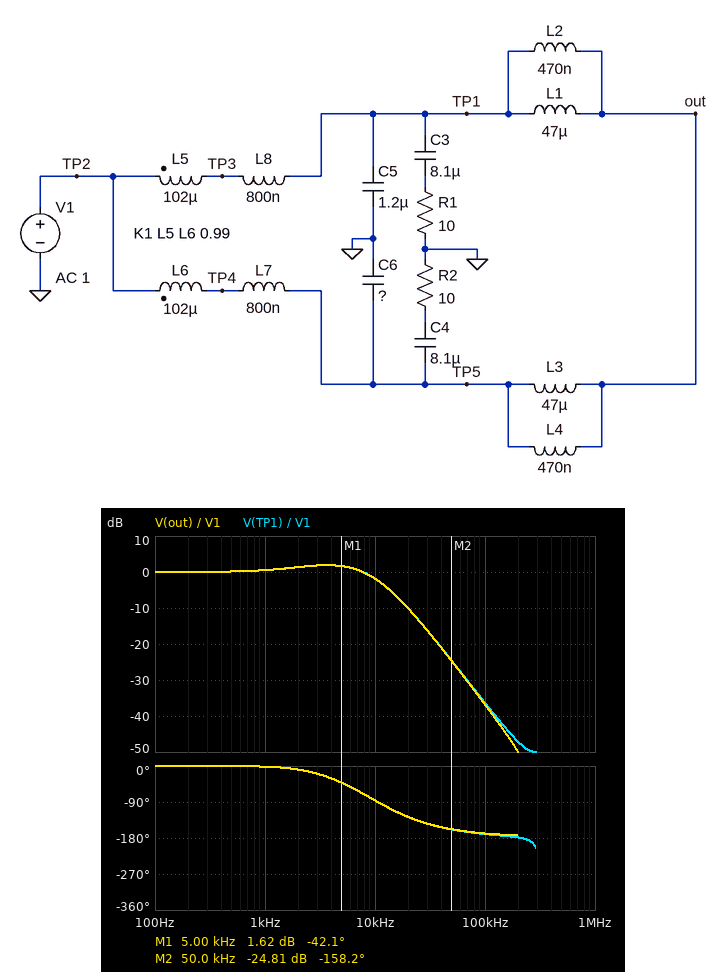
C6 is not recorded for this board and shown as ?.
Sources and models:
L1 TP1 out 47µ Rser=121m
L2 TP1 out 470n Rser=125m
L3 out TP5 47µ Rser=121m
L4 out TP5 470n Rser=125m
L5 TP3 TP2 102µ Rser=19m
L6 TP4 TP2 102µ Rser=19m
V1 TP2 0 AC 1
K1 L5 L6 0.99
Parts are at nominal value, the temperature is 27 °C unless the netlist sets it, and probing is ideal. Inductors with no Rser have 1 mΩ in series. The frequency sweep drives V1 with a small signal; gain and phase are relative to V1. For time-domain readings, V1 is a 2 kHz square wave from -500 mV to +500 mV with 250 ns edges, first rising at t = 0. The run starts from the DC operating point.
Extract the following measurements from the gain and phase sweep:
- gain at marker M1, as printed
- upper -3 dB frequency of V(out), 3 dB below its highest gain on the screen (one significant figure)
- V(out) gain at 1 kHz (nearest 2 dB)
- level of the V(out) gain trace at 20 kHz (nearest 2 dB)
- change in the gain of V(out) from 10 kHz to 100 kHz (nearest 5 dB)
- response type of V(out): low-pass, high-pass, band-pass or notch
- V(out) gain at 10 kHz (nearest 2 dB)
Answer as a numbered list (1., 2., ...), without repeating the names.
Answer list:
1. 1.62 dB
2. 9 kHz
3. 0 dB
4. -10 dB
5. -35 dB
6. low-pass
7. -2 dB
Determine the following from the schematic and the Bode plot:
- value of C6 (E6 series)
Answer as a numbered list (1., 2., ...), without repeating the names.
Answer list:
1. 470 nF
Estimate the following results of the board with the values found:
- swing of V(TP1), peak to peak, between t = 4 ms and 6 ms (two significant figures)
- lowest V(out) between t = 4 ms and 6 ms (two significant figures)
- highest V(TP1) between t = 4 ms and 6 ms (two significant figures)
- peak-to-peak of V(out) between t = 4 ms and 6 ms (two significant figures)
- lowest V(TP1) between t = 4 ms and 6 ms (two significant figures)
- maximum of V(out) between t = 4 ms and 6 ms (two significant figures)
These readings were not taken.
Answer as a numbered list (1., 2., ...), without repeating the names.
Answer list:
1. 1.4 V
2. -710 mV
3. 710 mV
4. 1.4 V
5. -710 mV
6. 710 mV
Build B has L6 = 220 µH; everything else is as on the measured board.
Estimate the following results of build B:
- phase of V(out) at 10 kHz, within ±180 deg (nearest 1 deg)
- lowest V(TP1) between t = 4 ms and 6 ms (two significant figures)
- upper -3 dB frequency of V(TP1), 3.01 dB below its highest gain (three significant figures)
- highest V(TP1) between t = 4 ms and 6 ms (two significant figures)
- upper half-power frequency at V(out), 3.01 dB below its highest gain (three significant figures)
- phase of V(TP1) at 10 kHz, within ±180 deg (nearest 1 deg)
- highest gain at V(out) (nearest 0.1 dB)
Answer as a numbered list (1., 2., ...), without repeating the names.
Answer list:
1. -32 deg
2. -530 mV
3. 26.9 kHz
4. 530 mV
5. 26.6 kHz
6. -29 deg
7. 0.5 dB
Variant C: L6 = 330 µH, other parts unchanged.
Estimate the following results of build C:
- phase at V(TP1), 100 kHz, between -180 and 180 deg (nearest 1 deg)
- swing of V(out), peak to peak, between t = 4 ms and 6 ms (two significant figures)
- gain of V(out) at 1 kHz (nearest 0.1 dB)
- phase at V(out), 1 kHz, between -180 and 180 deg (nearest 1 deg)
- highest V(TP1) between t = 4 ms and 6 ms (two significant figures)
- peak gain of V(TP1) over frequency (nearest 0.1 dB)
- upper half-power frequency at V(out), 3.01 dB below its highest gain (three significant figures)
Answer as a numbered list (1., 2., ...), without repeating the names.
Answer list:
1. -147 deg
2. 1.3 V
3. 0.2 dB
4. -3 deg
5. 670 mV
6. 2.0 dB
7. 38.5 kHz
